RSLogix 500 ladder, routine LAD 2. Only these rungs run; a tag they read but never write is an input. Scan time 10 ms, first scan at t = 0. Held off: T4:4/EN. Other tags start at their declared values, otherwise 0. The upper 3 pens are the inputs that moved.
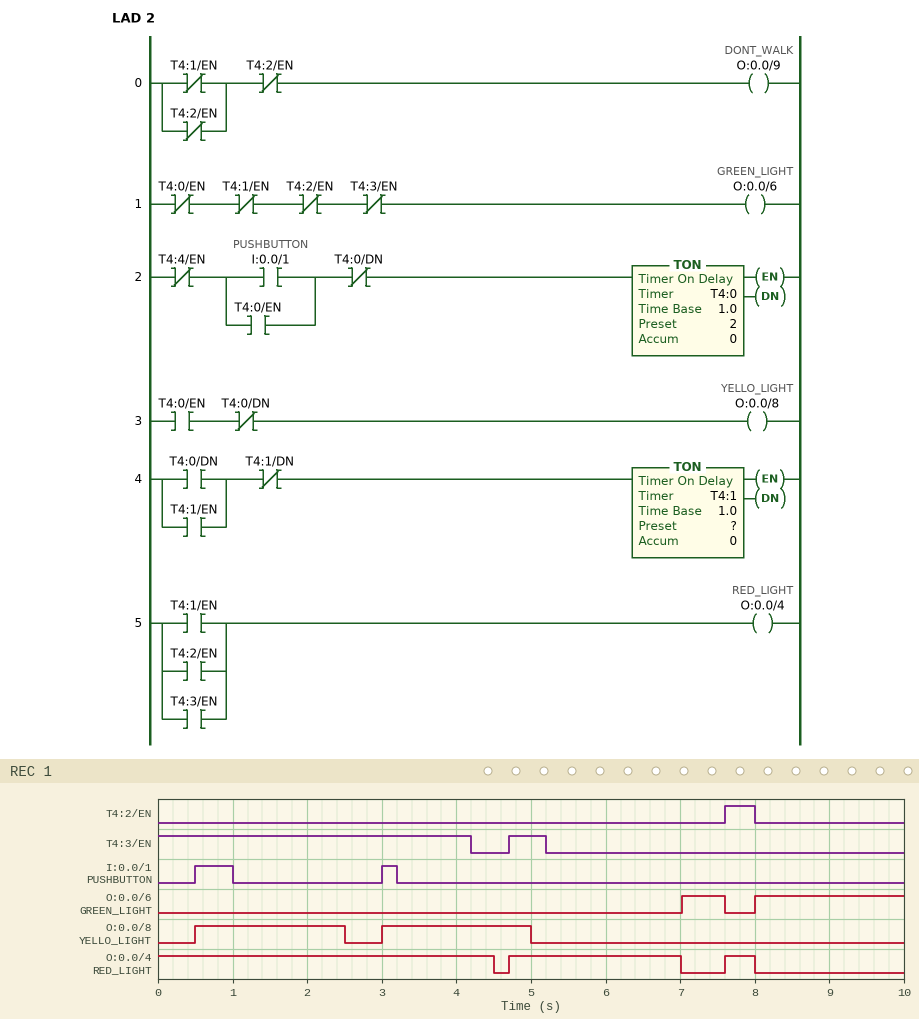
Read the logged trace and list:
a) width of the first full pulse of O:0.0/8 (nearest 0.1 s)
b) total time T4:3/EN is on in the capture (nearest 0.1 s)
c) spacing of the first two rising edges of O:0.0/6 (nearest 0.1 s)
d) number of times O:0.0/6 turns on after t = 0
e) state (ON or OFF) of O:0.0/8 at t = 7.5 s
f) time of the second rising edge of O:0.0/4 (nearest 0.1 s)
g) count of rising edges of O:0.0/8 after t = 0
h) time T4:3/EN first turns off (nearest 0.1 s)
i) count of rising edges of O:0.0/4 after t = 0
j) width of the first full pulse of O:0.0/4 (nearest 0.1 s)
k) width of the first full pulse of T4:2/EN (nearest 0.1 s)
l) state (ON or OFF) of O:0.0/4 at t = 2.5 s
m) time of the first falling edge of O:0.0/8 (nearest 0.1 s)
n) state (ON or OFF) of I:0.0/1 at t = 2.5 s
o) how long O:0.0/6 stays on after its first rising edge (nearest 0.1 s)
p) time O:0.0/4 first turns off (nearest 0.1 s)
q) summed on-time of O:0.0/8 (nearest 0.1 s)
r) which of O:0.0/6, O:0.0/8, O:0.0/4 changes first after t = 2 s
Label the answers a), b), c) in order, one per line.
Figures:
a) 2.0 s
b) 4.7 s
c) 1.0 s
d) 2
e) OFF
f) 7.6 s
g) 2
h) 4.2 s
i) 2
j) 2.3 s
k) 0.4 s
l) ON
m) 2.5 s
n) OFF
o) 0.6 s
p) 4.5 s
q) 4.0 s
r) O:0.0/8
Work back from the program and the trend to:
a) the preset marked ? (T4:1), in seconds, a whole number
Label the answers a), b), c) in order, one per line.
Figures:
a) 2 s
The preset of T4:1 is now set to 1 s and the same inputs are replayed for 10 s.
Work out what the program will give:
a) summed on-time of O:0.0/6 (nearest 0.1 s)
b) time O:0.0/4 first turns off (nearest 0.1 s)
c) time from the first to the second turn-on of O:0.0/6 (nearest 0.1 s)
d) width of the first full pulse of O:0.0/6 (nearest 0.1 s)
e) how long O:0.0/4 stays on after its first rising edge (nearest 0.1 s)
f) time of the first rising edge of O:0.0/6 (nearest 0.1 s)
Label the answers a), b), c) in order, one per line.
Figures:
a) 3.6 s
b) 4.2 s
c) 2.0 s
d) 1.6 s
e) 1.3 s
f) 6.0 s
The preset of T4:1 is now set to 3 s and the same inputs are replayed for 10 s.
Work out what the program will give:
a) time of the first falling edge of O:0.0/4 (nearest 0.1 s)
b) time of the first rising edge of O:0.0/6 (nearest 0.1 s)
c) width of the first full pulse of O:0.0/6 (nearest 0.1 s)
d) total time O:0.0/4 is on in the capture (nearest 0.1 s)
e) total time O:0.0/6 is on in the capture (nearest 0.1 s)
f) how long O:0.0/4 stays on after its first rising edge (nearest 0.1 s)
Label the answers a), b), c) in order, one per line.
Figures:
a) 5.5 s
b) 5.5 s
c) 2.1 s
d) 5.9 s
e) 4.1 s
f) 0.4 s
